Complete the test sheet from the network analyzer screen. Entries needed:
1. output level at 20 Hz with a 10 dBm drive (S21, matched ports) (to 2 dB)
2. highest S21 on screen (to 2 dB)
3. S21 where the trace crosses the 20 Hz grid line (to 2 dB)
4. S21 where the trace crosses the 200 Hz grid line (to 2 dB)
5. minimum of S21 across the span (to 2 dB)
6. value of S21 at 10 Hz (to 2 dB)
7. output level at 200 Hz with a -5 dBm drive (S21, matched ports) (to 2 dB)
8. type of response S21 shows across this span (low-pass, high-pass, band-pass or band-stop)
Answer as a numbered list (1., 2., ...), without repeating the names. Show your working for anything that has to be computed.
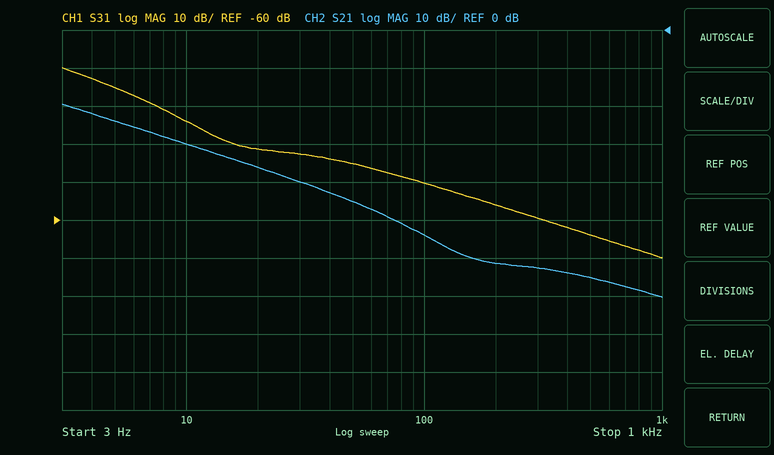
1. 10 dBm + (-36 dB) = -26 dBm
2. -20 dB
3. -36 dB
4. -62 dB
5. -70 dB
6. -30 dB
7. -5 dBm + (-62 dB) = -66 dBm
8. low-pass
